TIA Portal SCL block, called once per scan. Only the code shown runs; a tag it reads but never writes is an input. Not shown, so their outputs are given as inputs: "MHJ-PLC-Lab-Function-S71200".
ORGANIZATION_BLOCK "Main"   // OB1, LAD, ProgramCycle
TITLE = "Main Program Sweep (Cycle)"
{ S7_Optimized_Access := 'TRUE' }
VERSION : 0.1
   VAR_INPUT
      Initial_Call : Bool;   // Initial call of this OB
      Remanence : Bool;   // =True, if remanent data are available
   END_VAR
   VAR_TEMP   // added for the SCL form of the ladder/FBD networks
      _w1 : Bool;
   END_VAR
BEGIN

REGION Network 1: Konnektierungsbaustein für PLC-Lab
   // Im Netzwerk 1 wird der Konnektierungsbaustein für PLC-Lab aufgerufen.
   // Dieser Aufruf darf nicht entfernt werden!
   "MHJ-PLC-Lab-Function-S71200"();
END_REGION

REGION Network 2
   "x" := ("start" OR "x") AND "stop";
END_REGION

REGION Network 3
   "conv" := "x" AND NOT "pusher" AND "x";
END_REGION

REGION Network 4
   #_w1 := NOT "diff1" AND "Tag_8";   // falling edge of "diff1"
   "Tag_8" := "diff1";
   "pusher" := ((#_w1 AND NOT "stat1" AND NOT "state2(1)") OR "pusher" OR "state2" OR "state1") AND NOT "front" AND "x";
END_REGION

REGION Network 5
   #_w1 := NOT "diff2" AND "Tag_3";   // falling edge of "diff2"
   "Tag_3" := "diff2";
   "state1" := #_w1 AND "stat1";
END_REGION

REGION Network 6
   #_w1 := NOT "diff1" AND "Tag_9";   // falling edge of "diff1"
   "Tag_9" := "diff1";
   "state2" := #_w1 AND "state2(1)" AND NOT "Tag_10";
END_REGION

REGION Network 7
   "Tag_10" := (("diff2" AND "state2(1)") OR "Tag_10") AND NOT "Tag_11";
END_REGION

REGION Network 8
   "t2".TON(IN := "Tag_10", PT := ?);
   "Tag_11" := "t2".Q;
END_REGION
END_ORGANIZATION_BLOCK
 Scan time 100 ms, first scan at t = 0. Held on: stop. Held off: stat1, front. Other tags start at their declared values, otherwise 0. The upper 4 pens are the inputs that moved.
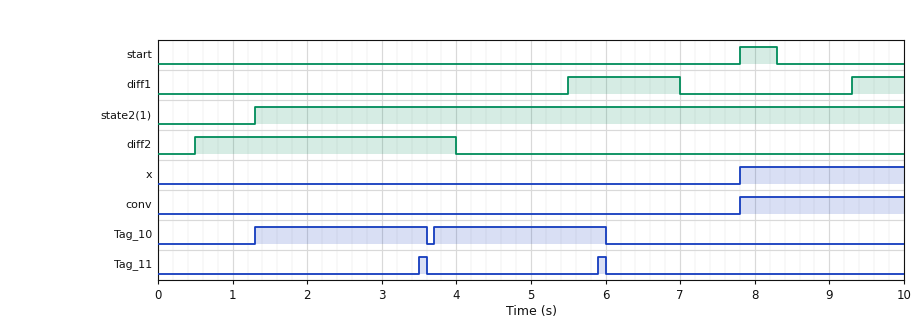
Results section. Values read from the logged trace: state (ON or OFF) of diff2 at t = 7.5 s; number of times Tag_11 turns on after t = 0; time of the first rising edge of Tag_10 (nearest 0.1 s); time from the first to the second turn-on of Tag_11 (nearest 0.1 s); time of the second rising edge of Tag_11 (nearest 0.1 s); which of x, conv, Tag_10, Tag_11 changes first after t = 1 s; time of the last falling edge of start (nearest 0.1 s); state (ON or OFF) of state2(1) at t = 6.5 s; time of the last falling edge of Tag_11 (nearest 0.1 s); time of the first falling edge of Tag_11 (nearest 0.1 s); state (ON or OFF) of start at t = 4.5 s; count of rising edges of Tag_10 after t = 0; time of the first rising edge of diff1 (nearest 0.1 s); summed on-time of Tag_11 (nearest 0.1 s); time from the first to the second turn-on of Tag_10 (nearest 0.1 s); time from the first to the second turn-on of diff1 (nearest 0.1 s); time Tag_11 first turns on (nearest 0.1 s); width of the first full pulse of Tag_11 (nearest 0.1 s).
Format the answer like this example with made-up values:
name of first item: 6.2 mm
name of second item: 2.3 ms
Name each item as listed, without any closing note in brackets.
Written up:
state (ON or OFF) of diff2 at t = 7.5 s: OFF
number of times Tag_11 turns on after t = 0: 2
time of the first rising edge of Tag_10: 1.3 s
time from the first to the second turn-on of Tag_11: 2.4 s
time of the second rising edge of Tag_11: 5.9 s
which of x, conv, Tag_10, Tag_11 changes first after t = 1 s: Tag_10
time of the last falling edge of start: 8.3 s
state (ON or OFF) of state2(1) at t = 6.5 s: ON
time of the last falling edge of Tag_11: 6.0 s
time of the first falling edge of Tag_11: 3.6 s
state (ON or OFF) of start at t = 4.5 s: OFF
count of rising edges of Tag_10 after t = 0: 2
time of the first rising edge of diff1: 5.5 s
summed on-time of Tag_11: 0.2 s
time from the first to the second turn-on of Tag_10: 2.4 s
time from the first to the second turn-on of diff1: 3.8 s
time Tag_11 first turns on: 3.5 s
width of the first full pulse of Tag_11: 0.1 s
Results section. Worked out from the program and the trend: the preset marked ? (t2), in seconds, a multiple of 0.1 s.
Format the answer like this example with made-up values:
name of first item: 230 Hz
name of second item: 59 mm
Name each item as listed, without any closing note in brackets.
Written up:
the preset marked ? (t2), in seconds, a multiple of 0.1 s: 2.2 s
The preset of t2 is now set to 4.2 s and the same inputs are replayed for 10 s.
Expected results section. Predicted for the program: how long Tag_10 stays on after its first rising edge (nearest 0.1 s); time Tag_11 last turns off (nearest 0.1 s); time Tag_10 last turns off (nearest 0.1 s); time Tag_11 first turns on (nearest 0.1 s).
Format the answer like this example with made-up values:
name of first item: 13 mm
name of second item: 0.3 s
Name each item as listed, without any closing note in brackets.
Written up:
how long Tag_10 stays on after its first rising edge: 4.3 s
time Tag_11 last turns off: 5.6 s
time Tag_10 last turns off: 5.6 s
time Tag_11 first turns on: 5.5 s
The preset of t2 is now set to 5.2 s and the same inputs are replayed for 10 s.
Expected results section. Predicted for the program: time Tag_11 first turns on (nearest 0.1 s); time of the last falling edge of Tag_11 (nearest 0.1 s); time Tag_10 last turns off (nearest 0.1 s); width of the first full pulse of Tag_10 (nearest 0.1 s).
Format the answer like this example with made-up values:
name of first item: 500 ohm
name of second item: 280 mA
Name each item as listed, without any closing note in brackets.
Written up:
time Tag_11 first turns on: 6.5 s
time of the last falling edge of Tag_11: 6.6 s
time Tag_10 last turns off: 6.6 s
width of the first full pulse of Tag_10: 5.3 s
